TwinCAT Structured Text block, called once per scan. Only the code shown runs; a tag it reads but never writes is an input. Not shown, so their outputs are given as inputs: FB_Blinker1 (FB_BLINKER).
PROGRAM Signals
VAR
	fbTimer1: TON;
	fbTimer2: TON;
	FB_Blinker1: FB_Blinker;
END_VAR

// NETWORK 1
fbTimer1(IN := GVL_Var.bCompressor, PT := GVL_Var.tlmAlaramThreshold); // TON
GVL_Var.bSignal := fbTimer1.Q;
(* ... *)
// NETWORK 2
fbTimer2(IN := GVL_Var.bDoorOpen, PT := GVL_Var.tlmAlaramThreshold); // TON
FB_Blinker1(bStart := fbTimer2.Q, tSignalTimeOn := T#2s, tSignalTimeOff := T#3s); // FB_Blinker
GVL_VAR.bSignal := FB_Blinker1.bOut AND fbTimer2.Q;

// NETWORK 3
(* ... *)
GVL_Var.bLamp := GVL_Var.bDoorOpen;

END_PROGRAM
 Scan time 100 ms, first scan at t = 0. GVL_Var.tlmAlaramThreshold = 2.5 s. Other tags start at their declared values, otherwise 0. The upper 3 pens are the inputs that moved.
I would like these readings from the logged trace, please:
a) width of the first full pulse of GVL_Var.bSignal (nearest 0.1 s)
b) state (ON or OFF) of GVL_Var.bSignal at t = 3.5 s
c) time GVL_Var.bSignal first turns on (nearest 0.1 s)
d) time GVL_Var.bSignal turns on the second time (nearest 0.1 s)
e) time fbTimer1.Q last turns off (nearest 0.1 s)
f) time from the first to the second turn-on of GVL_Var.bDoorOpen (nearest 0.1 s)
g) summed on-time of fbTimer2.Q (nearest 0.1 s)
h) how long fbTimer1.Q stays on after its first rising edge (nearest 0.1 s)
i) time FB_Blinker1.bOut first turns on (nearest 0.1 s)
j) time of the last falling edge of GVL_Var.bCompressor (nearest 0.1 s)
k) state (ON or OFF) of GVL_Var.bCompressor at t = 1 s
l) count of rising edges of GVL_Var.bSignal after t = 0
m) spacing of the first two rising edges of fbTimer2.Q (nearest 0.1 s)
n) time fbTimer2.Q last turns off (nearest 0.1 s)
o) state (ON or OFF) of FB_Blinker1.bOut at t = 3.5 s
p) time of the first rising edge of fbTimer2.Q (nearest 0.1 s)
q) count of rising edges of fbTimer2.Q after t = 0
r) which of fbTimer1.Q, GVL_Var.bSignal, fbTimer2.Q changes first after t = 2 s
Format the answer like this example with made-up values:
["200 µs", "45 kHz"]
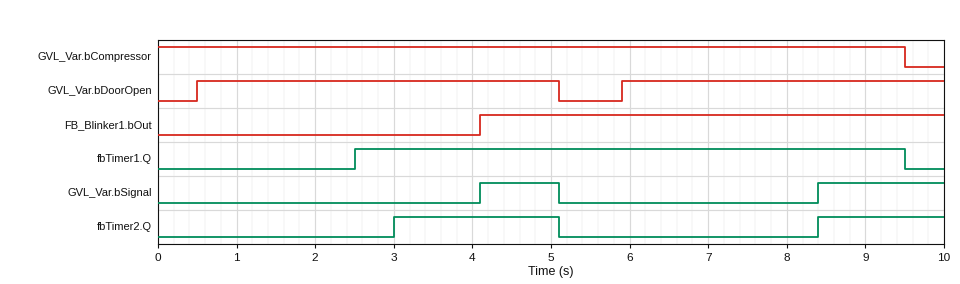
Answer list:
["1.0 s", "OFF", "4.1 s", "8.4 s", "9.5 s", "5.4 s", "3.7 s", "7.0 s", "4.1 s", "9.5 s", "ON", "2", "5.4 s", "5.1 s", "OFF", "3.0 s", "2", "fbTimer1.Q"]
